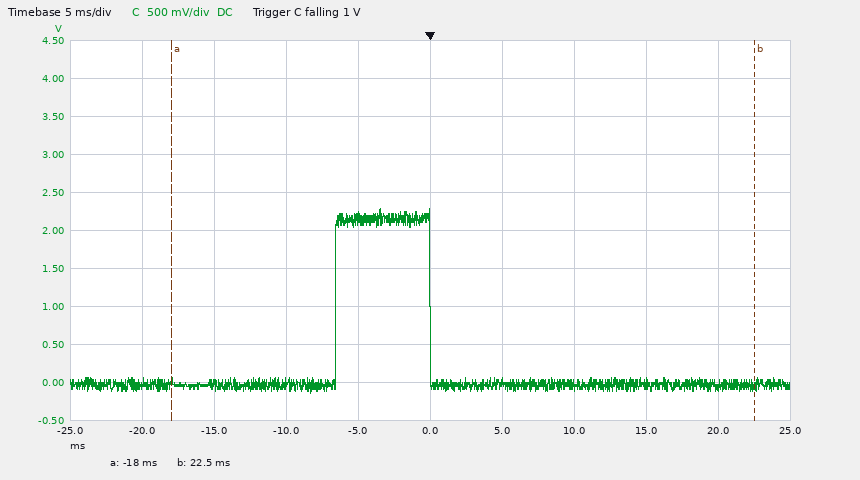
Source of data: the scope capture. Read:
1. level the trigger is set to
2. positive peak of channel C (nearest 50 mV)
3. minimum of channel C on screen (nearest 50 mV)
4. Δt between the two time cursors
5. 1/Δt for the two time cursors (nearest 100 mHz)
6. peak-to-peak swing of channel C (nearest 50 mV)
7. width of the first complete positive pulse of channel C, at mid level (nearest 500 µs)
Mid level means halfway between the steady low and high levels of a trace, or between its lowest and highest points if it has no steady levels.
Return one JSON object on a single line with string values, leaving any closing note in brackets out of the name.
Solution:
{"level the trigger is set to": "1 V", "positive peak of channel C": "2.30 V", "minimum of channel C on screen": "-150 mV", "Δt between the two time cursors": "40.5 ms", "1/Δt for the two time cursors": "24.7 Hz", "peak-to-peak swing of channel C": "2.45 V", "width of the first complete positive pulse of channel C, at mid level": "6.5 ms"}
